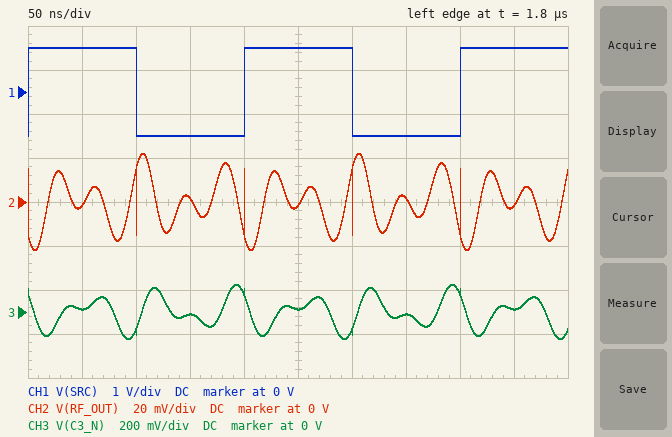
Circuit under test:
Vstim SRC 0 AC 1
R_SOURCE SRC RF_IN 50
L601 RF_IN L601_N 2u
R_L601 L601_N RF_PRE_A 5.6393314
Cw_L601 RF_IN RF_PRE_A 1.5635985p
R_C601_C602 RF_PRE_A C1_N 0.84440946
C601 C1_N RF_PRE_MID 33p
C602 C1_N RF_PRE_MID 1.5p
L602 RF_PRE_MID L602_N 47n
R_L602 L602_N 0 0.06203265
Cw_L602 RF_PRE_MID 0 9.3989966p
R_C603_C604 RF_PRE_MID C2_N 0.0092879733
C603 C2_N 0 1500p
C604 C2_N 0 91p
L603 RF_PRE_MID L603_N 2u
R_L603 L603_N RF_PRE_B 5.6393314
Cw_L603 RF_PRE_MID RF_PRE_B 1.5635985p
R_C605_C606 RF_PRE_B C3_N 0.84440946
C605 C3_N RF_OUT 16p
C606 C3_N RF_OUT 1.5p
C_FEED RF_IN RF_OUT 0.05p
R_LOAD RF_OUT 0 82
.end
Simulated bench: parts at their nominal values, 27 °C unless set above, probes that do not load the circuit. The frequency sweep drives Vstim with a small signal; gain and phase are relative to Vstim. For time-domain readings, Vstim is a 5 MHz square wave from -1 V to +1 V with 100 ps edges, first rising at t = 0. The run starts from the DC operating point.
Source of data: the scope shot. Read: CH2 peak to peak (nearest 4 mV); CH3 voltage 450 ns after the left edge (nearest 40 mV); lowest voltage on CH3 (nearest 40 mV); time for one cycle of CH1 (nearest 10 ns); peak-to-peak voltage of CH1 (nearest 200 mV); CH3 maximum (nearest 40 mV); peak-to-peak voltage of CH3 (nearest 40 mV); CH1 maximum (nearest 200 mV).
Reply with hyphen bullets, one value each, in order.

- 44 mV
- 0 V
- -120 mV
- 200 ns
- 2.0 V
- 120 mV
- 240 mV
- 1.0 V
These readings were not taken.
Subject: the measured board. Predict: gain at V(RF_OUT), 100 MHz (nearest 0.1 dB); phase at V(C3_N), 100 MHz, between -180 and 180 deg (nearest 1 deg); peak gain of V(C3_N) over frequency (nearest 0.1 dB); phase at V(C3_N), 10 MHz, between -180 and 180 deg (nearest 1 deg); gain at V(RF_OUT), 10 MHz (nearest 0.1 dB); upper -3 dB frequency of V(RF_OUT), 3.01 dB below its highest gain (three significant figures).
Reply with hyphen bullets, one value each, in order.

- -51.8 dB
- 88 deg
- 3.9 dB
- 167 deg
- -59.5 dB
- 20.0 MHz
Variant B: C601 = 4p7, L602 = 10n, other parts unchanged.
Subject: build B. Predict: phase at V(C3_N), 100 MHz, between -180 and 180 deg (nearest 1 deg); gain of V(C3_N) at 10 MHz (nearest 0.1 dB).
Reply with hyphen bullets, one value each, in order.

- 88 deg
- -69.8 dB
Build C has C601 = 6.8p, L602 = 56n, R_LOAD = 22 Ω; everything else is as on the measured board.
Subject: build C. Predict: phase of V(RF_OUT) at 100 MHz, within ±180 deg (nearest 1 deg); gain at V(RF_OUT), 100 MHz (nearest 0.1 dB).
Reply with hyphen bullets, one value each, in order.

- 89 deg
- -63.2 dB
